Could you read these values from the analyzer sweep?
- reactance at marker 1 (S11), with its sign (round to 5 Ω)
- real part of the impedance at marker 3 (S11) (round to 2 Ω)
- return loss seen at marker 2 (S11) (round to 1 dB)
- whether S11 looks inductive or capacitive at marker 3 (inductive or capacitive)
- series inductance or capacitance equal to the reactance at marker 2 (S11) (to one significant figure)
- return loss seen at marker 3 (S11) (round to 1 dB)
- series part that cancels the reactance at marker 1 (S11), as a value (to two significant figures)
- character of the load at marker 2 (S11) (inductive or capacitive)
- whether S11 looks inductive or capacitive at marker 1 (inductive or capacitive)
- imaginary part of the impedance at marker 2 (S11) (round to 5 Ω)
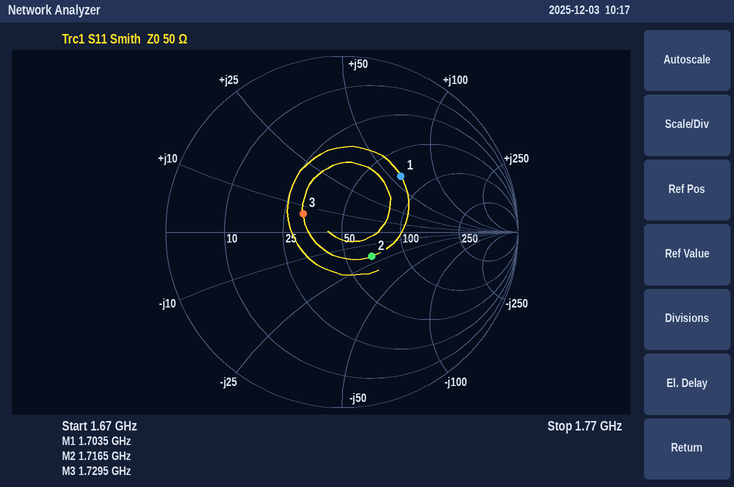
+60 Ω
32 Ω
13 dB
inductive
5 pF
12 dB
1.6 pF
capacitive
inductive
-20 Ω
